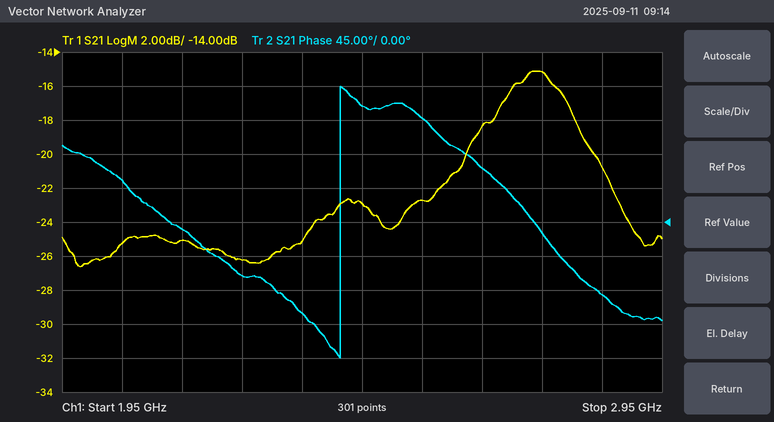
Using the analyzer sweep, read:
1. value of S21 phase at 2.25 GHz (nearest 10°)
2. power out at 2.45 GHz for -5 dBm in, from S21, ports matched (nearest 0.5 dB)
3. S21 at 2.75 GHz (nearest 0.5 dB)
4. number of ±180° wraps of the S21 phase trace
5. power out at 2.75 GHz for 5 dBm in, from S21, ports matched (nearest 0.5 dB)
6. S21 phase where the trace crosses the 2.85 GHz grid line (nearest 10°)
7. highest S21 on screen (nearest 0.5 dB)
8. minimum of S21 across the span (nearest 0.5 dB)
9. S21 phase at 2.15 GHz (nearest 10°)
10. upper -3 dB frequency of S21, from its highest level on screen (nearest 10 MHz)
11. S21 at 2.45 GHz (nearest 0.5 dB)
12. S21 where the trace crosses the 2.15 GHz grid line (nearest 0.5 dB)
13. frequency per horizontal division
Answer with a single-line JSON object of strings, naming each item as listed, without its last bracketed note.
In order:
{"value of S21 phase at 2.25 GHz": "-70°", "power out at 2.45 GHz for -5 dBm in, from S21, ports matched": "-28.0 dBm", "S21 at 2.75 GHz": "-15.0 dB", "number of ±180° wraps of the S21 phase trace": "1", "power out at 2.75 GHz for 5 dBm in, from S21, ports matched": "-10.0 dBm", "S21 phase where the trace crosses the 2.85 GHz grid line": "-100°", "highest S21 on screen": "-15.0 dB", "minimum of S21 across the span": "-26.5 dB", "S21 phase at 2.15 GHz": "-10°", "upper -3 dB frequency of S21, from its highest level on screen": "2.81 GHz", "S21 at 2.45 GHz": "-23.0 dB", "S21 where the trace crosses the 2.15 GHz grid line": "-25.0 dB", "frequency per horizontal division": "100 MHz"}
